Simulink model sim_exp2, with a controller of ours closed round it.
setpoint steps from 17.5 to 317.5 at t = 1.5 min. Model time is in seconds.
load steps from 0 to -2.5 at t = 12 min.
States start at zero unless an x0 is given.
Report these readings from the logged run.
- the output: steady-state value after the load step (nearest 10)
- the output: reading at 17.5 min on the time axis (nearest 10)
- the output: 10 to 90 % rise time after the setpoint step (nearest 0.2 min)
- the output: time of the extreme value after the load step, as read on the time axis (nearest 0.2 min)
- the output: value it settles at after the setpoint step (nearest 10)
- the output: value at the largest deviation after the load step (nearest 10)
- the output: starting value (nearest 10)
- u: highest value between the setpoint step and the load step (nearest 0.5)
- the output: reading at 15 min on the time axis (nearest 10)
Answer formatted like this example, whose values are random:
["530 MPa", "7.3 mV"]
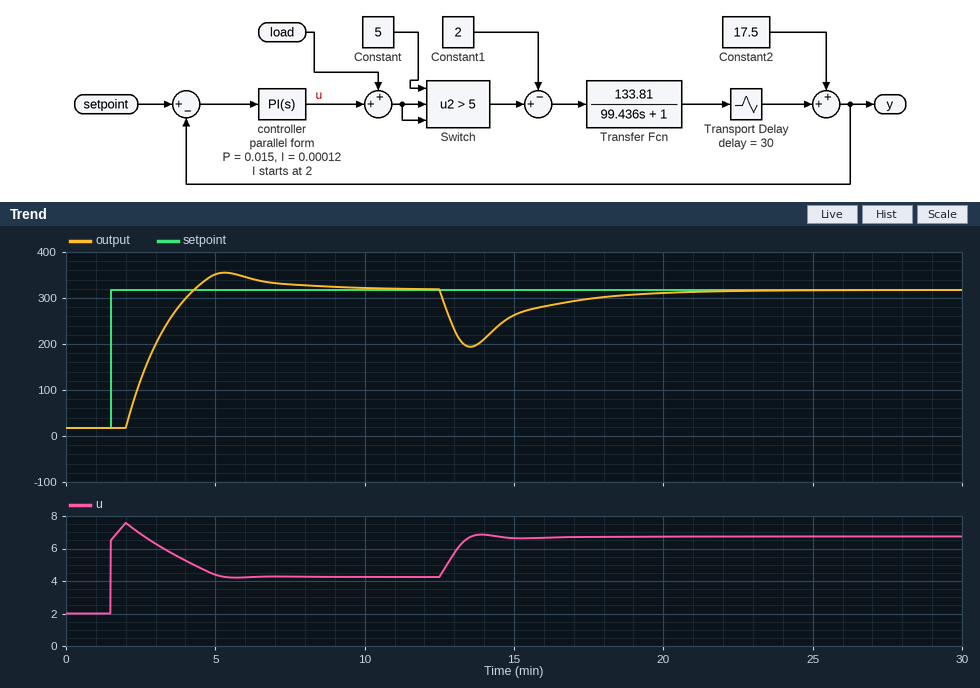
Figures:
["320", "300", "1.8 min", "13.6 min", "320", "190", "20", "7.5", "260"]
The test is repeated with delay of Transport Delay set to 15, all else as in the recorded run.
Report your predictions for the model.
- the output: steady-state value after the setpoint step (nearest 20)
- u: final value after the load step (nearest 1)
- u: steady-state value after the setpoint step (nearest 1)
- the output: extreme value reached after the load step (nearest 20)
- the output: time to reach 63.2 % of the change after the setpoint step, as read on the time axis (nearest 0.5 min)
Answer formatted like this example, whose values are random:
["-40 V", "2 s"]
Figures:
["320", "7", "4", "220", "3.0 min"]
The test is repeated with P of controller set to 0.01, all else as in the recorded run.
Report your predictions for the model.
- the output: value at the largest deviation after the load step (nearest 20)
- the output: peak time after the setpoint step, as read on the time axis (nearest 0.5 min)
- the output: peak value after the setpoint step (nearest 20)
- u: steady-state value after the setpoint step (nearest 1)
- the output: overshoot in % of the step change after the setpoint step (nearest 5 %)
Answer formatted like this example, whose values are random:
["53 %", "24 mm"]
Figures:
["180", "5.5 min", "360", "4", "15 %"]
